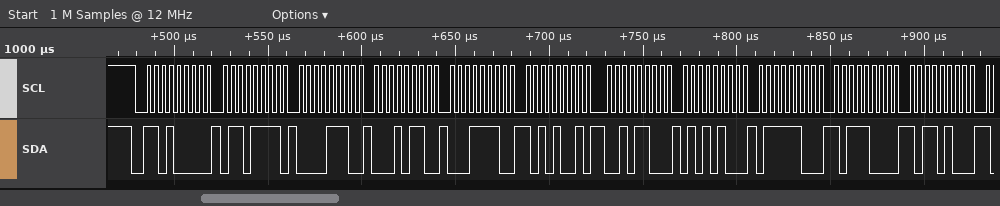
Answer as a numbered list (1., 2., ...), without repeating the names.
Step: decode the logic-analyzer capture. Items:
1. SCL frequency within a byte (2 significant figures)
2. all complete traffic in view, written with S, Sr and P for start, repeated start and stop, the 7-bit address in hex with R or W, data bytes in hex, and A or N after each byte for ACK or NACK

1. 250 kHz
2. S 68W A 6F A 0E A 16 A 1E A A9 A 2C A 54 A 7C A B8 A B4 A
